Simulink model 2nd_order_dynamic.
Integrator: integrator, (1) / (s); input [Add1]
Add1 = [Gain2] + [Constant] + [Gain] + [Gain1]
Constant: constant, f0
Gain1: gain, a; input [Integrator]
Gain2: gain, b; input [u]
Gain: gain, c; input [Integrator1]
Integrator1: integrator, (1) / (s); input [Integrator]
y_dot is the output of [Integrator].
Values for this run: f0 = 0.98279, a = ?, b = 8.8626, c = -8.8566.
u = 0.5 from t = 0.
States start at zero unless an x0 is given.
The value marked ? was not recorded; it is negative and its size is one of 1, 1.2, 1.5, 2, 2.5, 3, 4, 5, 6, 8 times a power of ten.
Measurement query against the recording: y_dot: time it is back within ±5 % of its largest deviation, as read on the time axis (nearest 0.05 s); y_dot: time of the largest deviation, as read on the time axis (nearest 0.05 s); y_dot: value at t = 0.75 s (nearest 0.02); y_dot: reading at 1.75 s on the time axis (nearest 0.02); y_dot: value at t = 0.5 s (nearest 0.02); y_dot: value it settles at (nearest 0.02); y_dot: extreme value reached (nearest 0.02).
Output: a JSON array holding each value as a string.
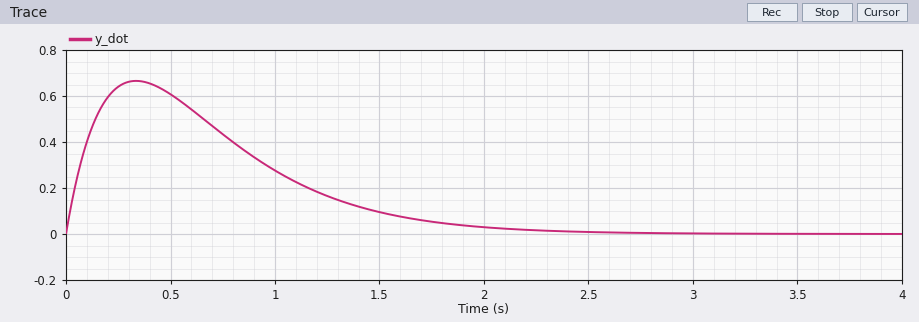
["1.95 s", "0.35 s", "0.44", "0.06", "0.60", "0.00", "0.66"]
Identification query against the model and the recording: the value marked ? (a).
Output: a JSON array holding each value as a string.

["-6"]
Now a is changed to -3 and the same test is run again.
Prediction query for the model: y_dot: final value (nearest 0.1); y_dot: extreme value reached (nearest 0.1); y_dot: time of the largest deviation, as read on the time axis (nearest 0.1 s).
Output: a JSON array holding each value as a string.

["0.0", "1.0", "0.4 s"]
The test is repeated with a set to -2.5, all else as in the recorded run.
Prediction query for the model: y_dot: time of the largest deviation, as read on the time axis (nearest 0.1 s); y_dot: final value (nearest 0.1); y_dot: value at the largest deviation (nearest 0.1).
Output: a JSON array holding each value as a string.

["0.4 s", "0.0", "1.1"]
